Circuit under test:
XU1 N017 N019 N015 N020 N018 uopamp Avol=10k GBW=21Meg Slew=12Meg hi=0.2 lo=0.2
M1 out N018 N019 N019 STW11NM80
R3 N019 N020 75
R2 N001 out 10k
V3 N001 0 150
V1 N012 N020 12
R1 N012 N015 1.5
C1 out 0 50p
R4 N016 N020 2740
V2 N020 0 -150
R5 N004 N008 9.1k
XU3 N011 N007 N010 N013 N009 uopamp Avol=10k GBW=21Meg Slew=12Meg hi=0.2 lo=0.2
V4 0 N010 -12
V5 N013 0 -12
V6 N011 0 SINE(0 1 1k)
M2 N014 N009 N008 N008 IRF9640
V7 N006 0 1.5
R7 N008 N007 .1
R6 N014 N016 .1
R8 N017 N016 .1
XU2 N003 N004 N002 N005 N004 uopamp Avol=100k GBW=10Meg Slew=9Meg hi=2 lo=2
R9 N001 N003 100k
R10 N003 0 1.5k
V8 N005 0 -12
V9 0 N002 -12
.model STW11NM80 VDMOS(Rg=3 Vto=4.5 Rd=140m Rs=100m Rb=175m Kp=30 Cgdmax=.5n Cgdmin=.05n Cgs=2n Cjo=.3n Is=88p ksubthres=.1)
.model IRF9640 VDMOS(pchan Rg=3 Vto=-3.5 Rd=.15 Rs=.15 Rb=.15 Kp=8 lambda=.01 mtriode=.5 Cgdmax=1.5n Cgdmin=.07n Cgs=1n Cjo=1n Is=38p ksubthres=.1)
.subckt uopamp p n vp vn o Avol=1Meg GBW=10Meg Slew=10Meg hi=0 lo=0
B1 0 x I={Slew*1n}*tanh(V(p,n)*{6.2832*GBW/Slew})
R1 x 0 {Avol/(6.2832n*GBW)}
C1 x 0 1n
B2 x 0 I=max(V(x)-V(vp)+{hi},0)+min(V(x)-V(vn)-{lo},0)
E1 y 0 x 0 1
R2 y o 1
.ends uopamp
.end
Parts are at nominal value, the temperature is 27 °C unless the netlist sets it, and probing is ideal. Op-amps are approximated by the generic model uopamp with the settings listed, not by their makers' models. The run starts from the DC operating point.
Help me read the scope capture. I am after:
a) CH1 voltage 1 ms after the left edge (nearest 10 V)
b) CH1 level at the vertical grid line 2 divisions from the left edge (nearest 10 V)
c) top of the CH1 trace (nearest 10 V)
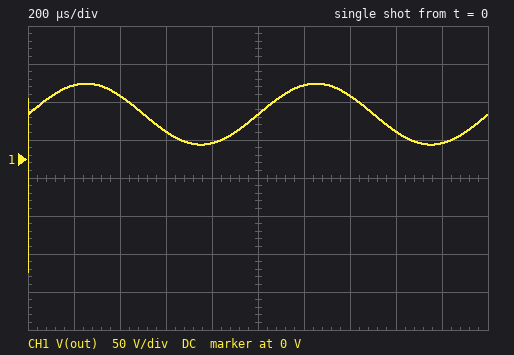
60 V
80 V
100 V
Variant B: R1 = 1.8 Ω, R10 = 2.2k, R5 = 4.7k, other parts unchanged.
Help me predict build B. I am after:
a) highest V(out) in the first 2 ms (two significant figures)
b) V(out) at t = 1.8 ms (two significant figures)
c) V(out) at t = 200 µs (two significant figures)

-25 V
-150 V
-29 V
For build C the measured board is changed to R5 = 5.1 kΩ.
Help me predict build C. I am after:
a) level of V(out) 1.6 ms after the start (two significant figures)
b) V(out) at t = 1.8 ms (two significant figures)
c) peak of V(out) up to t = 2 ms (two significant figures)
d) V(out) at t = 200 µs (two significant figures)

-52 V
-79 V
61 V
57 V
